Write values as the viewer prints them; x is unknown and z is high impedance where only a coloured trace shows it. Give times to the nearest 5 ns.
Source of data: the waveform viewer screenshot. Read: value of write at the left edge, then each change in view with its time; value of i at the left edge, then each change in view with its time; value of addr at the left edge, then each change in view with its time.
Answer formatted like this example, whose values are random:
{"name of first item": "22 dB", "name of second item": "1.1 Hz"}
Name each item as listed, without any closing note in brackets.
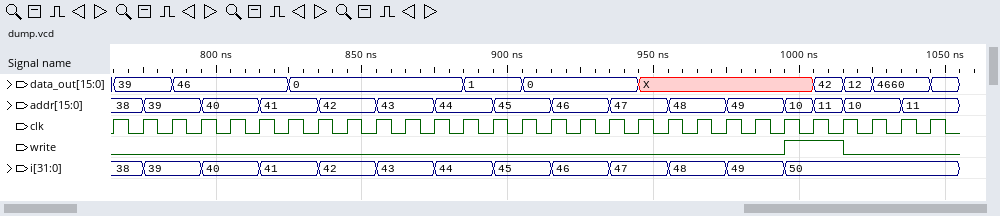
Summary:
{"value of write at the left edge, then each change in view with its time": "0, 1 at 995 ns, 0 at 1015 ns", "value of i at the left edge, then each change in view with its time": "38, 39 at 775 ns, 40 at 795 ns, 41 at 815 ns, 42 at 835 ns, 43 at 855 ns, 44 at 875 ns, 45 at 895 ns, 46 at 915 ns, 47 at 935 ns, 48 at 955 ns, 49 at 975 ns, 50 at 995 ns", "value of addr at the left edge, then each change in view with its time": "38, 39 at 775 ns, 40 at 795 ns, 41 at 815 ns, 42 at 835 ns, 43 at 855 ns, 44 at 875 ns, 45 at 895 ns, 46 at 915 ns, 47 at 935 ns, 48 at 955 ns, 49 at 975 ns, 10 at 995 ns, 11 at 1005 ns, 10 at 1015 ns, 11 at 1035 ns"}
